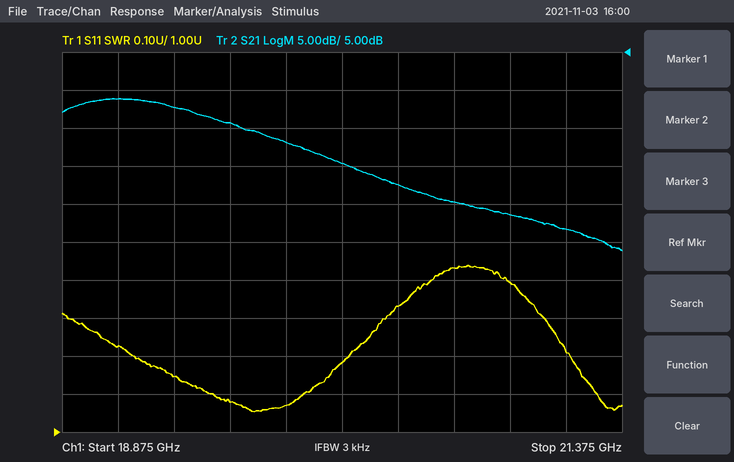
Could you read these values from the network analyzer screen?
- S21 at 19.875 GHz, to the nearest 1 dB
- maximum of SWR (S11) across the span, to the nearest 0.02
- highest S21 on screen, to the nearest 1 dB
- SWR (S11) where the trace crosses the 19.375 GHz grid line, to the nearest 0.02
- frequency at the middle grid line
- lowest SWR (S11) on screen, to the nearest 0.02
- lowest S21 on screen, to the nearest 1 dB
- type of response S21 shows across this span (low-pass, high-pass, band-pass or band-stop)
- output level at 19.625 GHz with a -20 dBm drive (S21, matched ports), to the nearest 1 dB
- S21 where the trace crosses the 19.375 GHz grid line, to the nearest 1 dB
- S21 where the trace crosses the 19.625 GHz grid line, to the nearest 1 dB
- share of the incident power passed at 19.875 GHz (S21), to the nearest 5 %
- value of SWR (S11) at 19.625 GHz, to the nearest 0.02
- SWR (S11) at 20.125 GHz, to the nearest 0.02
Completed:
-7 dB
1.44
-1 dB
1.14
20.125 GHz
1.06
-21 dB
low-pass
-24 dBm
-2 dB
-4 dB
20 %
1.08
1.18
